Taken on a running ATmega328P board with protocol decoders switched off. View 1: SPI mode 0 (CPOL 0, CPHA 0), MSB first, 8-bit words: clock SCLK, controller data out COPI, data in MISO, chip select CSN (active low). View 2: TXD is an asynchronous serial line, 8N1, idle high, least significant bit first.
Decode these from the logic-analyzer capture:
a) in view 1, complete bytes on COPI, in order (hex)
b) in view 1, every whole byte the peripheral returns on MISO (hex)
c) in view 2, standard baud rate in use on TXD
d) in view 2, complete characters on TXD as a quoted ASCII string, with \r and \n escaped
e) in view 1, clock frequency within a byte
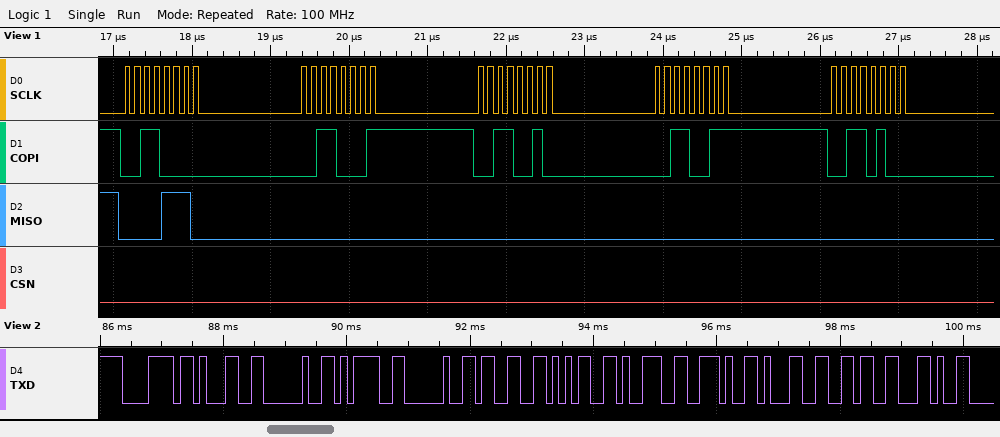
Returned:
0x30 0x31 0x32 0x33 0x34
0x0E 0x00 0x00 0x00 0x00
9600 baud
"x1 = 359.16,"
8 MHz
